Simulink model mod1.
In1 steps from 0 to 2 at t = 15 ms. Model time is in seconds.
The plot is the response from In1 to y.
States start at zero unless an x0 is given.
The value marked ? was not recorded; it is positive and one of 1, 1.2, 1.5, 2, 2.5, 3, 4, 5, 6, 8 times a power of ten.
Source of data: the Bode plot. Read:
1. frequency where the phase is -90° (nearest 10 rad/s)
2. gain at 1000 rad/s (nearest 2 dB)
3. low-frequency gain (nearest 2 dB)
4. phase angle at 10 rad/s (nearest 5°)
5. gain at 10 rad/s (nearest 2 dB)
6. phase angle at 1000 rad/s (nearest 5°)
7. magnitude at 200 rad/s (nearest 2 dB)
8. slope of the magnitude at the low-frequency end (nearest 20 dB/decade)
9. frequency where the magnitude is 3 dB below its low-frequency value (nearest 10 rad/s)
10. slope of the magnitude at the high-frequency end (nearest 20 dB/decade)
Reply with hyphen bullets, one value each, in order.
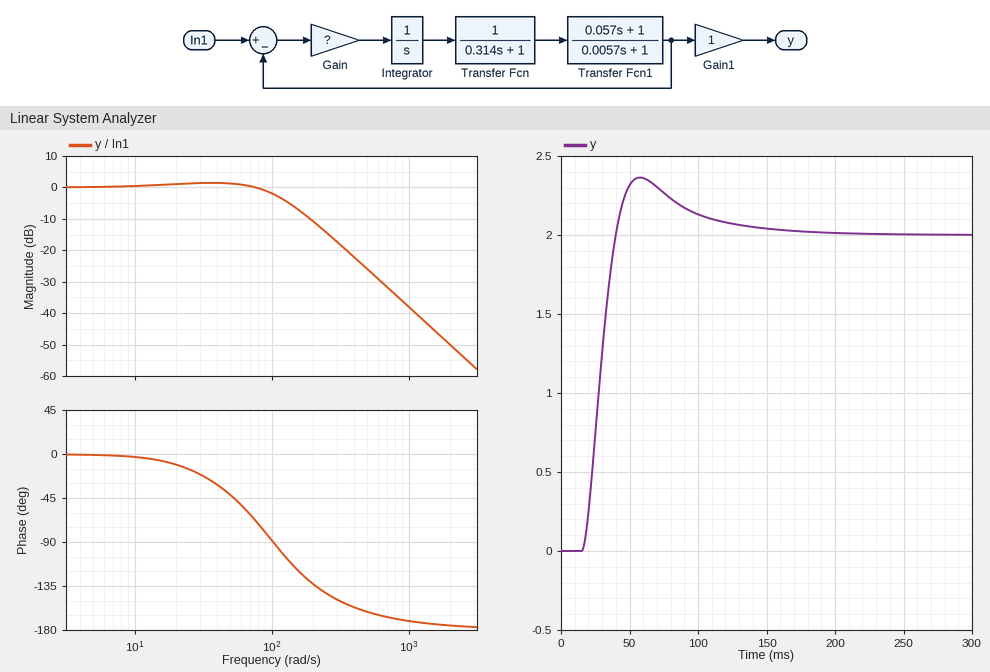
- 100 rad/s
- -38 dB
- 0 dB
- -5°
- 0 dB
- -170°
- -10 dB
- 0 dB/decade
- 110 rad/s
- -40 dB/decade
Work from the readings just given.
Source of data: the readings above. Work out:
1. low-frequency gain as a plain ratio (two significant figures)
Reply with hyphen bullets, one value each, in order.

- 1.0
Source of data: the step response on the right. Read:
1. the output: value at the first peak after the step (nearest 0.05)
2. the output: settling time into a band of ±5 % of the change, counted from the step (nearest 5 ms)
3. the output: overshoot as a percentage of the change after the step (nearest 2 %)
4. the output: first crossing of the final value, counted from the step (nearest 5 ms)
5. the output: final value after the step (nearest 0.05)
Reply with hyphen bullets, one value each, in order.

- 2.35
- 95 ms
- 18 %
- 25 ms
- 2.00
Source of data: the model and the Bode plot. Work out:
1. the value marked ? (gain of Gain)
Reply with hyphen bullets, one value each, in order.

- 400
